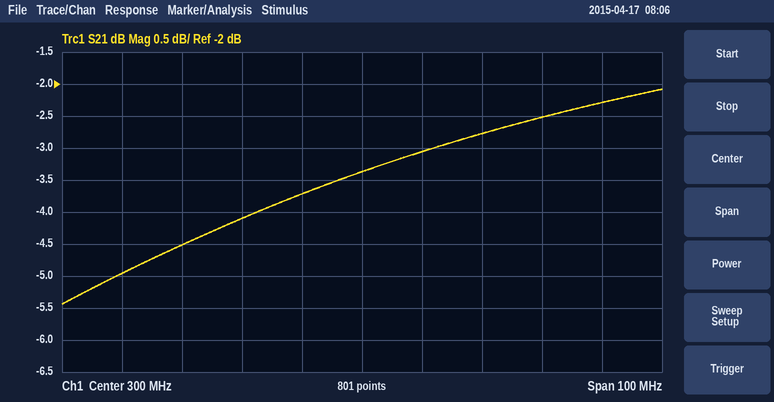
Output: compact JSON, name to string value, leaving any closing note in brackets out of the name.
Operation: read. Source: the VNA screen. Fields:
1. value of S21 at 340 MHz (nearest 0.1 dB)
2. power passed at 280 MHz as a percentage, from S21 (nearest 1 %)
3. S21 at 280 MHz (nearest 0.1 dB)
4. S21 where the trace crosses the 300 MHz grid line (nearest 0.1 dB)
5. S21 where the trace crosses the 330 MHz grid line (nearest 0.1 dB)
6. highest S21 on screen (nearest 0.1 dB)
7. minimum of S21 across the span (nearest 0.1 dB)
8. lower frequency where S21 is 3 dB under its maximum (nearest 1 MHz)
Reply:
{"value of S21 at 340 MHz": "-2.3 dB", "power passed at 280 MHz as a percentage, from S21": "39 %", "S21 at 280 MHz": "-4.1 dB", "S21 where the trace crosses the 300 MHz grid line": "-3.4 dB", "S21 where the trace crosses the 330 MHz grid line": "-2.5 dB", "highest S21 on screen": "-2.1 dB", "minimum of S21 across the span": "-5.4 dB", "lower frequency where S21 is 3 dB under its maximum": "257 MHz"}
